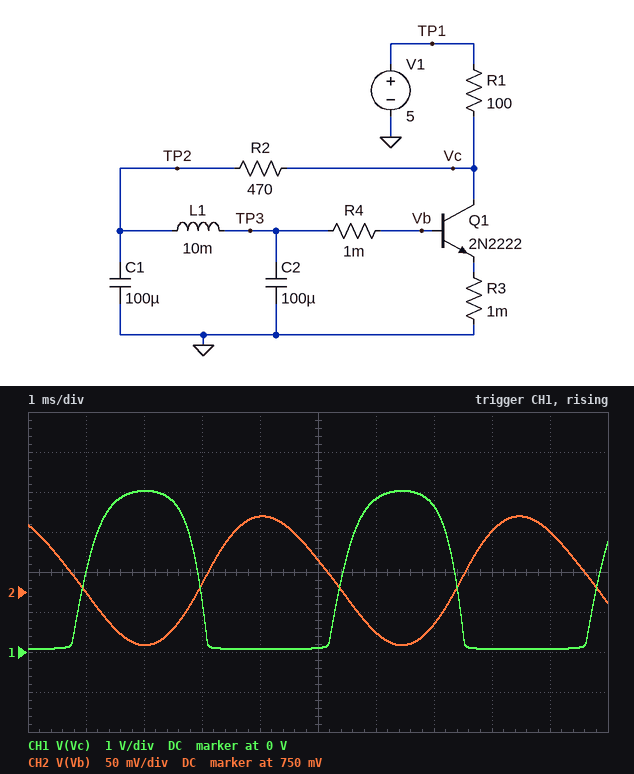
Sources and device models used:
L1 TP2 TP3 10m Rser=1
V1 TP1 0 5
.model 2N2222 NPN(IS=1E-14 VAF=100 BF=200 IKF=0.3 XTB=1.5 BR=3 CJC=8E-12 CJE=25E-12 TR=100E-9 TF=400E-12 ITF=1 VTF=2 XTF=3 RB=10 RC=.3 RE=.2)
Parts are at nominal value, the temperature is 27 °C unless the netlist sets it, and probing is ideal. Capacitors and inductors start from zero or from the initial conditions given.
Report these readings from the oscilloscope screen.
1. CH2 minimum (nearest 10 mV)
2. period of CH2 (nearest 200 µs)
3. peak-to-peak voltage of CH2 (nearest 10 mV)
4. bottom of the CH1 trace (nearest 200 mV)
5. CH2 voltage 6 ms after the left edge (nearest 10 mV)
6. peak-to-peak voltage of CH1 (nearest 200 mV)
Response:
680 mV
4.4 ms
160 mV
0 V
700 mV
4.0 V
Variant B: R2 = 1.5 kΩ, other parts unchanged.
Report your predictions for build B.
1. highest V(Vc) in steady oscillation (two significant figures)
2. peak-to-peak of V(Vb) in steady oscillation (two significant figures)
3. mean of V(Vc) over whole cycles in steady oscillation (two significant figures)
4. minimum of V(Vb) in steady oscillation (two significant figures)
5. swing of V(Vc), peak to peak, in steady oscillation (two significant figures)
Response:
3.2 V
54 mV
1.4 V
730 mV
3.1 V
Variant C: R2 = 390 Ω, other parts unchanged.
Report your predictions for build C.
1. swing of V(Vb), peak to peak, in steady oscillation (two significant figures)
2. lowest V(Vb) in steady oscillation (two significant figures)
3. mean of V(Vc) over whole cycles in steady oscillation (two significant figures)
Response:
190 mV
670 mV
1.7 V
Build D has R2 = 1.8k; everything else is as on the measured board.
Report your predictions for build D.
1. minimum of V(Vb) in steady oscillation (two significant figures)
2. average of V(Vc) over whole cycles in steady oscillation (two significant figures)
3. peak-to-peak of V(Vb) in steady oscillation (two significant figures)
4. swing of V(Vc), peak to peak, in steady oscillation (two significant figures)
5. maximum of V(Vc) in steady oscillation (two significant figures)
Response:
740 mV
1.4 V
46 mV
2.9 V
3.0 V
